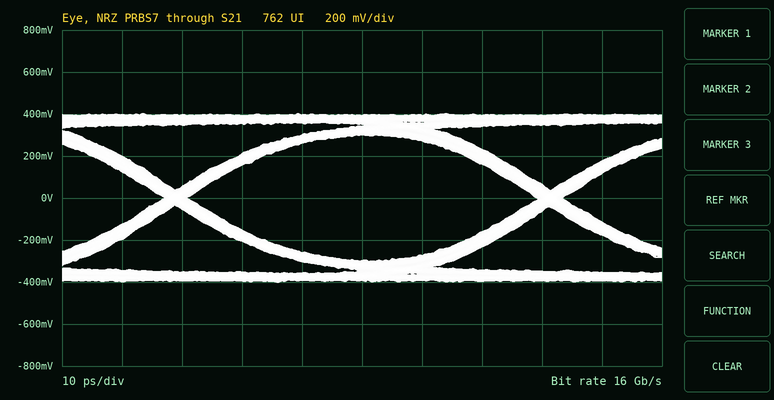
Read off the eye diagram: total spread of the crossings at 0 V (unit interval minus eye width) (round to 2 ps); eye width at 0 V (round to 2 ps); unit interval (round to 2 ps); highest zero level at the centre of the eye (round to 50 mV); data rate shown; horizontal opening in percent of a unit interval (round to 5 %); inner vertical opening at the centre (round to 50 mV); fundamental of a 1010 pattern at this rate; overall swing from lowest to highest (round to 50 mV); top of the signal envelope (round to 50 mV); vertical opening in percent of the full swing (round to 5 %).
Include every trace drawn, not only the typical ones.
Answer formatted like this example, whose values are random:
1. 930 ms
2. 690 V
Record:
1. 4 ps
2. 58 ps
3. 62 ps
4. -300 mV
5. 16 Gb/s
6. 95 %
7. 600 mV
8. 8 GHz
9. 800 mV
10. 400 mV
11. 75 %
